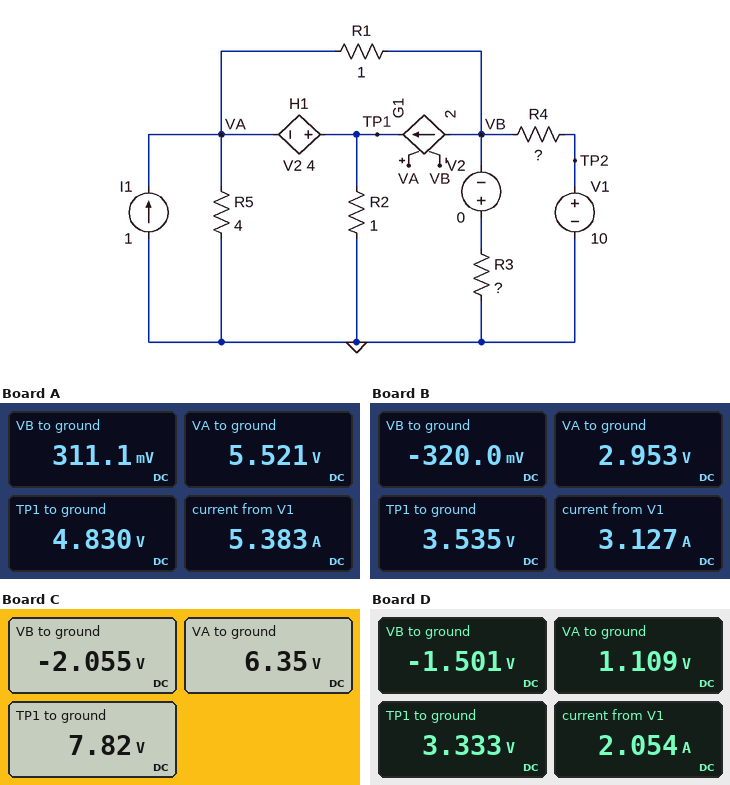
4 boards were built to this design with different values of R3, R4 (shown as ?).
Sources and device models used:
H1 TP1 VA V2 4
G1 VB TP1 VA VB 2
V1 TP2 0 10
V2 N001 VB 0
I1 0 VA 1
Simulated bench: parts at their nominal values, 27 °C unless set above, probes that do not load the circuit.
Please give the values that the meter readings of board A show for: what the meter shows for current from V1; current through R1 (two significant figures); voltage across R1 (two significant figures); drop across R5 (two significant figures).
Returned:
5.383 A
5.2 A
5.2 V
5.5 V
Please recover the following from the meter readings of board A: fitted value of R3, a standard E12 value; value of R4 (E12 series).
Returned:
1.8 Ω
1.8 Ω
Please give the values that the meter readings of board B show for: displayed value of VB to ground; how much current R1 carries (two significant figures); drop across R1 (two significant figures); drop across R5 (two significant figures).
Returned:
-320.0 mV
3.3 A
3.3 V
3.0 V
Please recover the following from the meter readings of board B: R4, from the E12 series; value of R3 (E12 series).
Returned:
3.3 Ω
2.2 Ω
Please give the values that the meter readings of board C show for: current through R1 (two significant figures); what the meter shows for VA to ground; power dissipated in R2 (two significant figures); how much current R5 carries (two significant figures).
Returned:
8.4 A
6.35 V
61 W
1.6 A
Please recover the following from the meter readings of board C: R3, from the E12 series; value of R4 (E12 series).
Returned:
5.6 Ω
1.5 Ω
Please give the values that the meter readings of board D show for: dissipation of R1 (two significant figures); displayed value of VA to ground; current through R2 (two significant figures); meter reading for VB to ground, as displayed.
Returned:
6.8 W
1.109 V
3.3 A
-1.501 V
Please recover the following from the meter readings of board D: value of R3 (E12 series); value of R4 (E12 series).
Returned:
2.7 Ω
5.6 Ω
